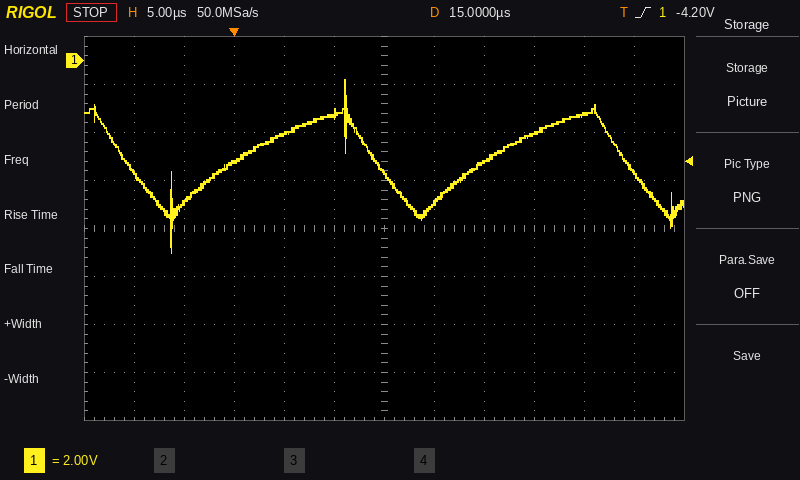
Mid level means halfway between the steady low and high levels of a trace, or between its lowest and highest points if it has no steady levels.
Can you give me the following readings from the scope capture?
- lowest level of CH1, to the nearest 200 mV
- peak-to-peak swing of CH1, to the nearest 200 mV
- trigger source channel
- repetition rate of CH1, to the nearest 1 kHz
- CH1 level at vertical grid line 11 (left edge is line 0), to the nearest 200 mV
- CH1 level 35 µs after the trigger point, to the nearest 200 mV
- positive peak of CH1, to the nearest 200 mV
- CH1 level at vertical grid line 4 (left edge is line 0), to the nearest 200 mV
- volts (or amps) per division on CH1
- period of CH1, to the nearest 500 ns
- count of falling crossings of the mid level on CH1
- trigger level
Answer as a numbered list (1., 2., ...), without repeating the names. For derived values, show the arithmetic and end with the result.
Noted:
1. -8.0 V
2. -800 mV − (-8.0 V) = 7.2 V
3. CH1
4. 1 / 25.0 µs ≈ 40 kHz
5. -4.6 V
6. -2.2 V
7. -800 mV
8. -3.0 V
9. 2 V
10. 25.0 µs
11. 3
12. -4.20 V
